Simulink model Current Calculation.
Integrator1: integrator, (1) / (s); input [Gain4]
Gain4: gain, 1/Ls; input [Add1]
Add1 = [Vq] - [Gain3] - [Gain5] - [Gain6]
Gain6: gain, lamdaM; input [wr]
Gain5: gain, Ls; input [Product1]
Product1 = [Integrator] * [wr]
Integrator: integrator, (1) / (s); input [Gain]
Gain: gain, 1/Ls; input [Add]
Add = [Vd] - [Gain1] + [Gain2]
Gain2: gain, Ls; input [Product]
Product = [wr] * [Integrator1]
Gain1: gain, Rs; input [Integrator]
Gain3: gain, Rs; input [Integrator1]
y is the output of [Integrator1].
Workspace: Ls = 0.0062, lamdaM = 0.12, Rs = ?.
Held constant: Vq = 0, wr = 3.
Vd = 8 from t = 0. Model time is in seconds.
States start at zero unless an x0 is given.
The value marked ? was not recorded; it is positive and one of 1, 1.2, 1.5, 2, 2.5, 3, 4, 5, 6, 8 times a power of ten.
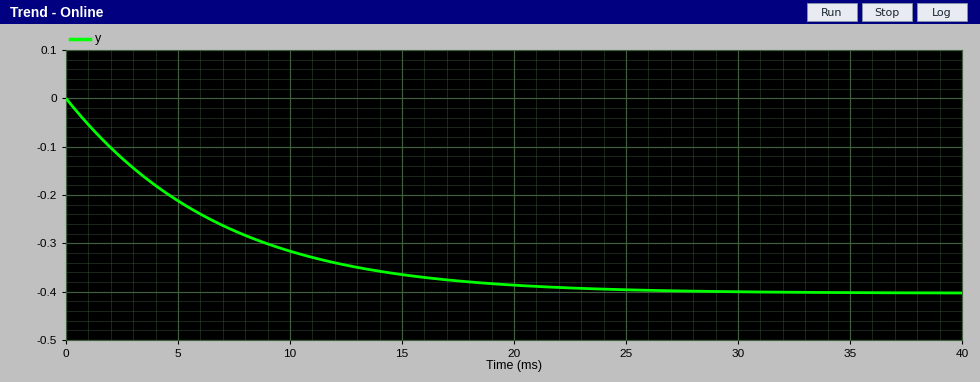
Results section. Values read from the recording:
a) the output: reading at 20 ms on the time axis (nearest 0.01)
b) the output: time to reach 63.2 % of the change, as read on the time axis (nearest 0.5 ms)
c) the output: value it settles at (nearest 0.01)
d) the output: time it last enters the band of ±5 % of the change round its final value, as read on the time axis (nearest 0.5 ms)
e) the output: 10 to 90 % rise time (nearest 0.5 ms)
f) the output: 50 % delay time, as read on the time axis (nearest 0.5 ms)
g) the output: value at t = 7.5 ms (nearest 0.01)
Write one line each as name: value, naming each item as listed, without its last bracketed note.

the output: reading at 20 ms on the time axis: -0.39
the output: time to reach 63.2 % of the change, as read on the time axis: 6.5 ms
the output: value it settles at: -0.40
the output: time it last enters the band of ±5 % of the change round its final value, as read on the time axis: 19.0 ms
the output: 10 to 90 % rise time: 14.0 ms
the output: 50 % delay time, as read on the time axis: 4.5 ms
the output: value at t = 7.5 ms: -0.27
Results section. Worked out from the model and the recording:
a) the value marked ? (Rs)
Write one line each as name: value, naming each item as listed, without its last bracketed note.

the value marked ?: 1.2
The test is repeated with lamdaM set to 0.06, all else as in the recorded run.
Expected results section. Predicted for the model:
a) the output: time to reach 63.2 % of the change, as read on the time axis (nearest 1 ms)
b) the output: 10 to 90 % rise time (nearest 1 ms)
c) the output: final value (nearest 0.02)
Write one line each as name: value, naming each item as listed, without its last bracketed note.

the output: time to reach 63.2 % of the change, as read on the time axis: 8 ms
the output: 10 to 90 % rise time: 15 ms
the output: final value: -0.26
